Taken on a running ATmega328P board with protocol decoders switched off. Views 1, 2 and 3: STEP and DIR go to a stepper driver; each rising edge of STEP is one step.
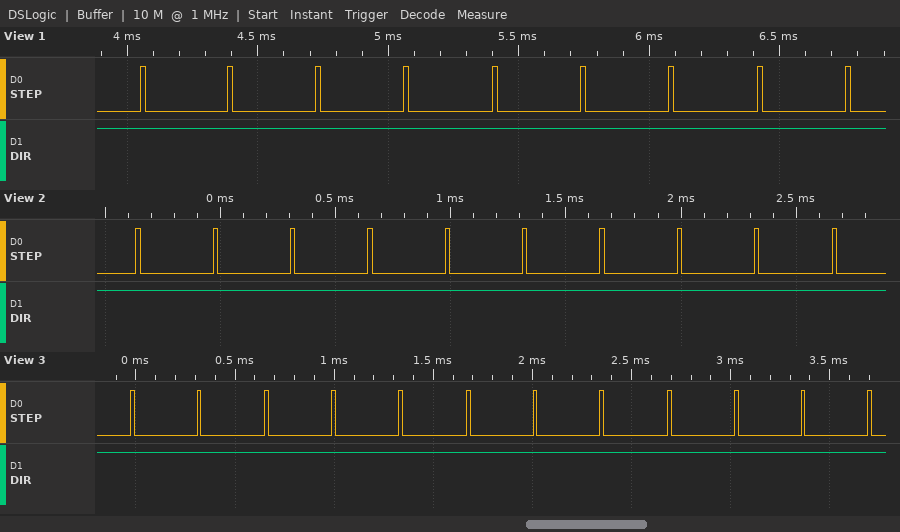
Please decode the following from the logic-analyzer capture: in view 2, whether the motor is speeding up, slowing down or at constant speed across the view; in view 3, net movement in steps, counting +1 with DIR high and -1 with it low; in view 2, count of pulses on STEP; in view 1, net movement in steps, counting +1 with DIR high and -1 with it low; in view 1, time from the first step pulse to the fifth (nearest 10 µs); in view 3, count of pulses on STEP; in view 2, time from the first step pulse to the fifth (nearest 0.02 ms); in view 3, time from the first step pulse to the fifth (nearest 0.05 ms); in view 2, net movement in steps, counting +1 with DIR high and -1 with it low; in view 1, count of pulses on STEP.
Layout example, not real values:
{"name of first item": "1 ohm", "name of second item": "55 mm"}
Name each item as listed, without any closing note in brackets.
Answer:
{"in view 2, whether the motor is speeding up, slowing down or at constant speed across the view": "constant speed", "in view 3, net movement in steps, counting +1 with DIR high and -1 with it low": "+12", "in view 2, count of pulses on STEP": "10", "in view 1, net movement in steps, counting +1 with DIR high and -1 with it low": "+9", "in view 1, time from the first step pulse to the fifth": "1350 µs", "in view 3, count of pulses on STEP": "12", "in view 2, time from the first step pulse to the fifth": "1.34 ms", "in view 3, time from the first step pulse to the fifth": "1.35 ms", "in view 2, net movement in steps, counting +1 with DIR high and -1 with it low": "+10", "in view 1, count of pulses on STEP": "9"}
